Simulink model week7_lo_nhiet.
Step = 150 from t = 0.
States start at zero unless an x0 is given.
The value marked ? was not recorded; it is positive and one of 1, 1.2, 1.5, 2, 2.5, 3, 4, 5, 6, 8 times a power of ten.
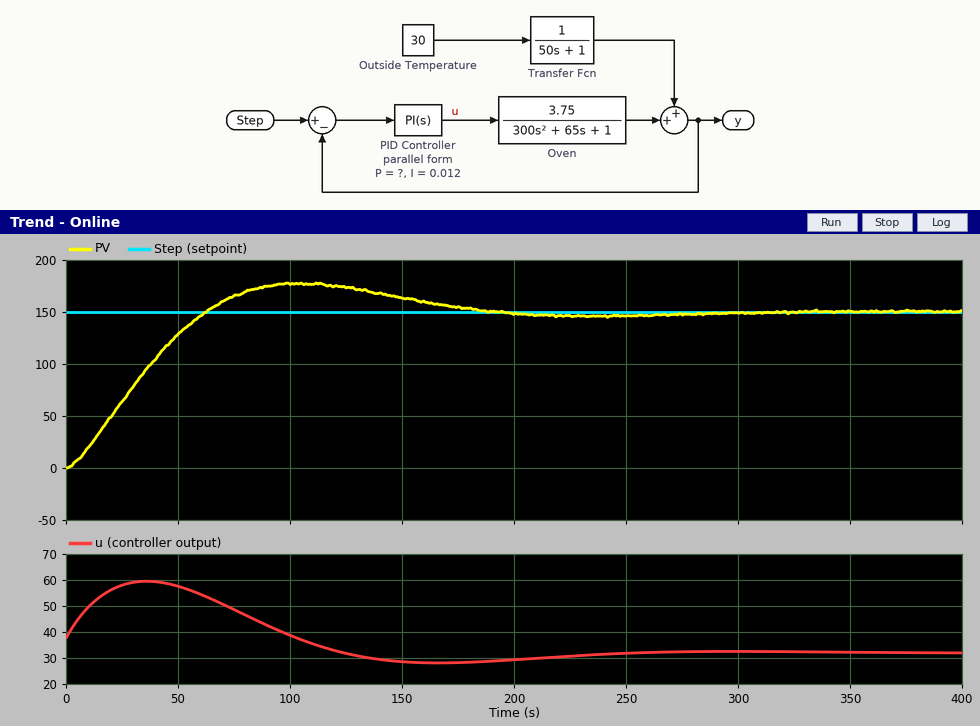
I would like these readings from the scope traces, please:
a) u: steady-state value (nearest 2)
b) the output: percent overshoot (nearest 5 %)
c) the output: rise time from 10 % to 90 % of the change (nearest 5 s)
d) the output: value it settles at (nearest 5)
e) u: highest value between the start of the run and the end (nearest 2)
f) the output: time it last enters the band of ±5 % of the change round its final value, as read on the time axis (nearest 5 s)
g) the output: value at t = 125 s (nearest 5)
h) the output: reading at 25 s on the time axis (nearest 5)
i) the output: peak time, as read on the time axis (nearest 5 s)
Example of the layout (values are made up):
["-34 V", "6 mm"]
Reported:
["32", "20 %", "45 s", "150", "60", "165 s", "175", "65", "105 s"]
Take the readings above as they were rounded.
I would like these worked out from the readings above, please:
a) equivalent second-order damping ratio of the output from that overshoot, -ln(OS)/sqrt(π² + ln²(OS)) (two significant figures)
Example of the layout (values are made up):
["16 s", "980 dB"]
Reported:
["0.46"]
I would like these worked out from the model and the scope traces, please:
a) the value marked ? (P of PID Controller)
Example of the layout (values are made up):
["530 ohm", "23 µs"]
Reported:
["0.25"]
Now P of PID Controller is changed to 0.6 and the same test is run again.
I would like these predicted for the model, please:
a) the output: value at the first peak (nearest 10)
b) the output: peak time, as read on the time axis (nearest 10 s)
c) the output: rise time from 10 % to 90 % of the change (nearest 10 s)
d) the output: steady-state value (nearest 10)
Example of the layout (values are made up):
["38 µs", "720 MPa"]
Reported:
["160", "90 s", "40 s", "150"]
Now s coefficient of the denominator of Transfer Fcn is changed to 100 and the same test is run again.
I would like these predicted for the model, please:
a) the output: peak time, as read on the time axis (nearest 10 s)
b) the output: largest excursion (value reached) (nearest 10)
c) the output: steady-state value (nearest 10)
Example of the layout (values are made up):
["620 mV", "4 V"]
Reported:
["110 s", "180", "150"]
